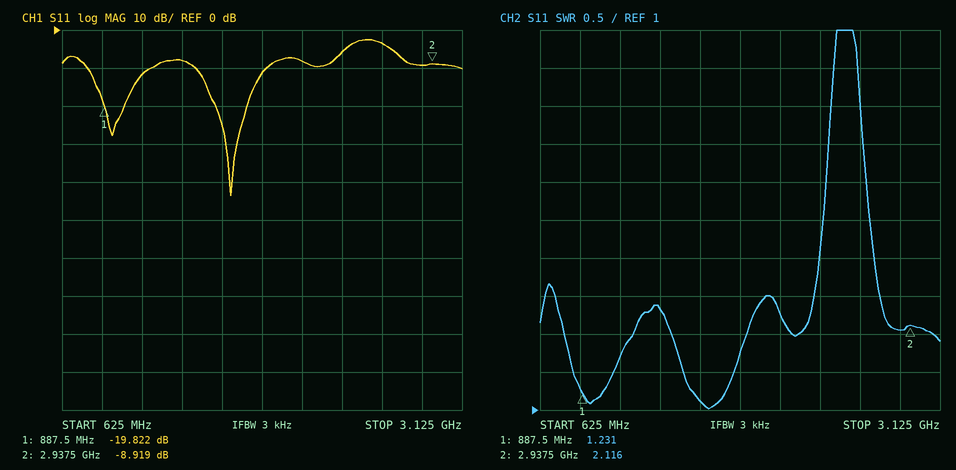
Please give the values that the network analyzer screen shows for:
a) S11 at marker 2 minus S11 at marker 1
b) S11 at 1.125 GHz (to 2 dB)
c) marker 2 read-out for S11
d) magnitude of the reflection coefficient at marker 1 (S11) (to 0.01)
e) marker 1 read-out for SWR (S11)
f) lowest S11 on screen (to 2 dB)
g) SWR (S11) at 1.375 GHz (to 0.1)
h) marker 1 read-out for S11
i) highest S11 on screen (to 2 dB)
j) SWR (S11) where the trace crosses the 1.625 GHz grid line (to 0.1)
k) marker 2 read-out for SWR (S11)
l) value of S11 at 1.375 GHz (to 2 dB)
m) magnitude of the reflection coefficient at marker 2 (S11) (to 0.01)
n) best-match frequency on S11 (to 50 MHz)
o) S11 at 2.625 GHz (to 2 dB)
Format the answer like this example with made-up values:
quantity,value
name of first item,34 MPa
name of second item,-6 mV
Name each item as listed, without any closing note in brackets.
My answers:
quantity,value
S11 at marker 2 minus S11 at marker 1,10.903 dB
S11 at 1.125 GHz,-12 dB
marker 2 read-out for S11,-8.919 dB
magnitude of the reflection coefficient at marker 1 (S11),0.10
marker 1 read-out for SWR,1.231
lowest S11 on screen,-44 dB
SWR (S11) at 1.375 GHz,2.3
marker 1 read-out for S11,-19.822 dB
highest S11 on screen,-2 dB
SWR (S11) where the trace crosses the 1.625 GHz grid line,1.1
marker 2 read-out for SWR,2.116
value of S11 at 1.375 GHz,-8 dB
magnitude of the reflection coefficient at marker 2 (S11),0.36
best-match frequency on S11,1.70 GHz
S11 at 2.625 GHz,-4 dB
